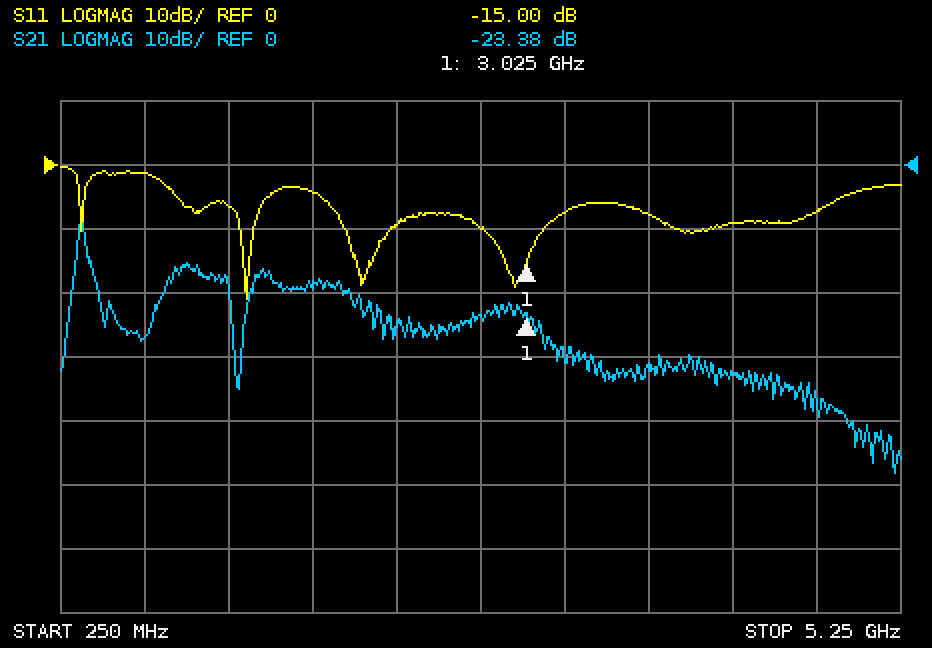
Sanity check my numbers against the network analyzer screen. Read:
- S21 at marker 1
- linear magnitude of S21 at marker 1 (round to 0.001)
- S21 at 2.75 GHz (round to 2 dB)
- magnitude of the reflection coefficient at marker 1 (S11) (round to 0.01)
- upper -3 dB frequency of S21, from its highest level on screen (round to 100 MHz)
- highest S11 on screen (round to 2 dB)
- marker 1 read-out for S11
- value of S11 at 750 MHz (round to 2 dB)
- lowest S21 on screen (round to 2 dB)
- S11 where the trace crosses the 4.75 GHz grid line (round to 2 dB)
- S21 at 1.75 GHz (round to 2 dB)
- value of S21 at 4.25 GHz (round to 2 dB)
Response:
-23.38 dB
0.068
-24 dB
0.18
400 MHz
0 dB
-15.00 dB
-2 dB
-48 dB
-8 dB
-18 dB
-32 dB
